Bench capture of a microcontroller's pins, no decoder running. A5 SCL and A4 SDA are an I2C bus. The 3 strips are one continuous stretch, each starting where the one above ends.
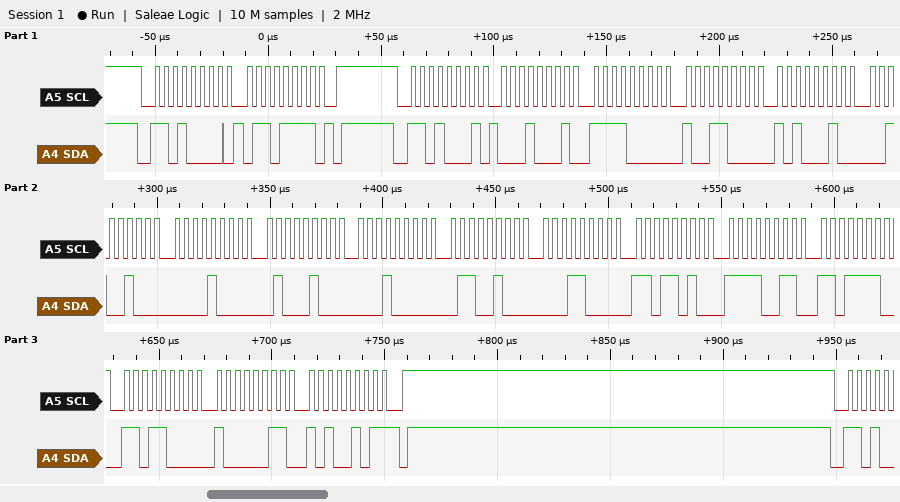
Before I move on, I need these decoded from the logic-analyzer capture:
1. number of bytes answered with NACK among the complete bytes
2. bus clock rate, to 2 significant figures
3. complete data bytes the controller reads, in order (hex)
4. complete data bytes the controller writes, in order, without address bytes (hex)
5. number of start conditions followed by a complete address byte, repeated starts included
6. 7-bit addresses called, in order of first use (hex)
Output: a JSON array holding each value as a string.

["1", "250 kHz", "11 F0 98 A2 24 08 44 10 64 18 DA F3 DE D8 83 A5", "6F", "2", "0x68"]
